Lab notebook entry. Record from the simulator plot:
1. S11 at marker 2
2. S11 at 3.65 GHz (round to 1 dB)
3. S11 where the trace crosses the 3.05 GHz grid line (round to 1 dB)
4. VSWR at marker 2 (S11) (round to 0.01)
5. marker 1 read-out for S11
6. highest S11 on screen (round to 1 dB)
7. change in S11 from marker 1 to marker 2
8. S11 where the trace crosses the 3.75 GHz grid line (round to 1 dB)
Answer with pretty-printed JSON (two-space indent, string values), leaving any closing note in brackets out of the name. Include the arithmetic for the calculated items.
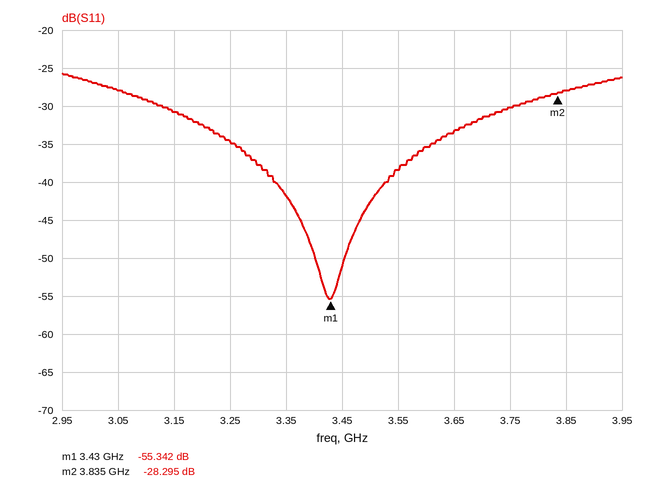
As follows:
{
  "S11 at marker 2": "-28.295 dB",
  "S11 at 3.65 GHz": "-33 dB",
  "S11 where the trace crosses the 3.05 GHz grid line": "-28 dB",
  "VSWR at marker 2 (S11)": "(1 + 0.0385)/(1 − 0.0385) ≈ 1.08",
  "marker 1 read-out for S11": "-55.342 dB",
  "highest S11 on screen": "-26 dB",
  "change in S11 from marker 1 to marker 2": "-28.295 − (-55.342) = 27.047 dB",
  "S11 where the trace crosses the 3.75 GHz grid line": "-30 dB"
}
